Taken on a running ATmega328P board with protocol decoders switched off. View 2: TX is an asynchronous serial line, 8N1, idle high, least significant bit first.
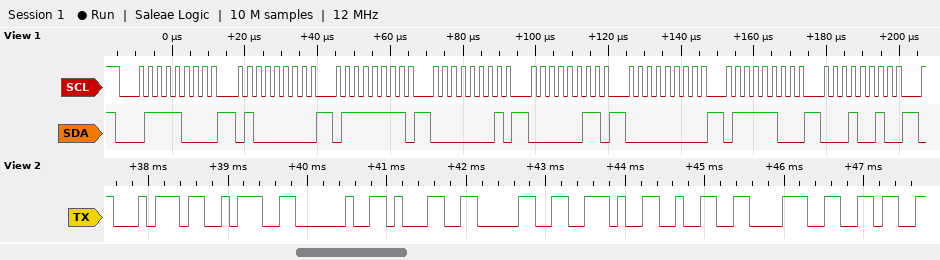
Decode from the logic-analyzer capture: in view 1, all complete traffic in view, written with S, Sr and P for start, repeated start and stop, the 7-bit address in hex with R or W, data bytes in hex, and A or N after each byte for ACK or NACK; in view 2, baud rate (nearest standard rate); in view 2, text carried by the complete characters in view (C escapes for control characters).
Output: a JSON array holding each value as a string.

["S 3CW A 40 A 7F A 01 A 03 A 00 A 7C A 12 A", "9600 baud", "\"t: 10.286\""]
